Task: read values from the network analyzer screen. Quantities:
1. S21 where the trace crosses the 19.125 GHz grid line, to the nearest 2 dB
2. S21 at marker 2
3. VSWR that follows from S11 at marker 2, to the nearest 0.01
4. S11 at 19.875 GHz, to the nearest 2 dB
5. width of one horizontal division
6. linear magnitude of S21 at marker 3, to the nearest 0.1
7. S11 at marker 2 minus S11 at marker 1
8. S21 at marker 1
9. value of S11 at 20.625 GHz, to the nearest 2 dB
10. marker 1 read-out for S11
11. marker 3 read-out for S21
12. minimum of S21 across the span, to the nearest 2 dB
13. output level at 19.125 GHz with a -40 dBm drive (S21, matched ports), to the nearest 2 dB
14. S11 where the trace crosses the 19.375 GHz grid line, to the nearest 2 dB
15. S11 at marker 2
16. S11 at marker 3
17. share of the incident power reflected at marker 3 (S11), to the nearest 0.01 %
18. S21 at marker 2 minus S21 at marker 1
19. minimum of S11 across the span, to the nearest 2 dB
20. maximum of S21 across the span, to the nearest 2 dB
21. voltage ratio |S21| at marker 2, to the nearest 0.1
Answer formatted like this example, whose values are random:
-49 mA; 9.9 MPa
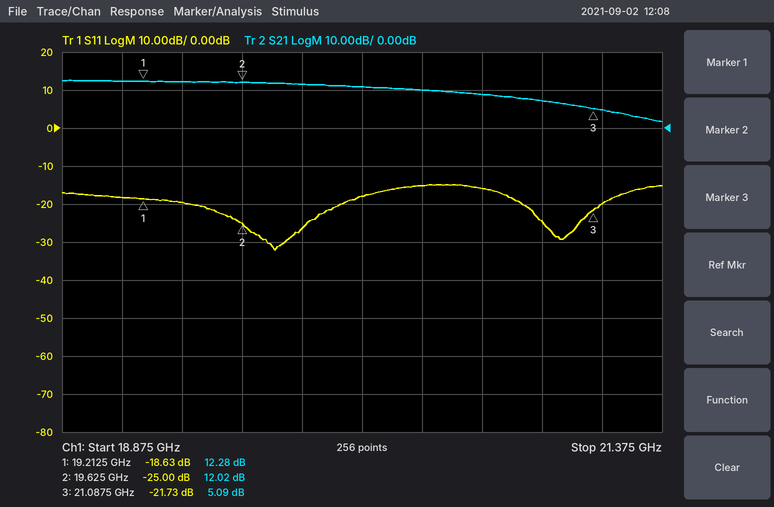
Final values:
12 dB; 12.02 dB; 1.12; -26 dB; 250 MHz; 1.8; -6.37 dB; 12.28 dB; -16 dB; -18.63 dB; 5.09 dB; 2 dB; -28 dBm; -20 dB; -25.00 dB; -21.73 dB; 0.67 %; -0.26 dB; -32 dB; 12 dB; 4.0
